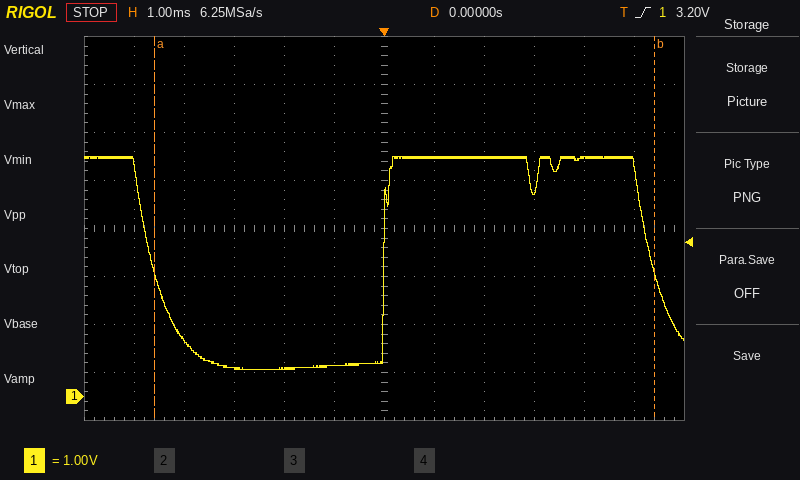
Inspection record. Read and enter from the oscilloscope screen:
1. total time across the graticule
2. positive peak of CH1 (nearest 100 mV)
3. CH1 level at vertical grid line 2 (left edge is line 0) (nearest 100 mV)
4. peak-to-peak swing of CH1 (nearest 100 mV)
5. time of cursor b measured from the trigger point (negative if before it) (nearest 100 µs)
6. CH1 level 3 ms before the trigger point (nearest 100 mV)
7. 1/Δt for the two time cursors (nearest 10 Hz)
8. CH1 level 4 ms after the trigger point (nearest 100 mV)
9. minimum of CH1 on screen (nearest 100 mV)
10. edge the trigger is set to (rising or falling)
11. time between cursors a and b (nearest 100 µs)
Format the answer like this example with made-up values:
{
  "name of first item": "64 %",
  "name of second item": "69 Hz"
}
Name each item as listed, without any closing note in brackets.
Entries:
{
  "total time across the graticule": "12 ms",
  "positive peak of CH1": "5.0 V",
  "CH1 level at vertical grid line 2 (left edge is line 0)": "1.2 V",
  "peak-to-peak swing of CH1": "4.4 V",
  "time of cursor b measured from the trigger point (negative if before it)": "+5.4 ms",
  "CH1 level 3 ms before the trigger point": "600 mV",
  "1/Δt for the two time cursors": "100 Hz",
  "CH1 level 4 ms after the trigger point": "5.0 V",
  "minimum of CH1 on screen": "600 mV",
  "edge the trigger is set to": "rising",
  "time between cursors a and b": "10.0 ms"
}
